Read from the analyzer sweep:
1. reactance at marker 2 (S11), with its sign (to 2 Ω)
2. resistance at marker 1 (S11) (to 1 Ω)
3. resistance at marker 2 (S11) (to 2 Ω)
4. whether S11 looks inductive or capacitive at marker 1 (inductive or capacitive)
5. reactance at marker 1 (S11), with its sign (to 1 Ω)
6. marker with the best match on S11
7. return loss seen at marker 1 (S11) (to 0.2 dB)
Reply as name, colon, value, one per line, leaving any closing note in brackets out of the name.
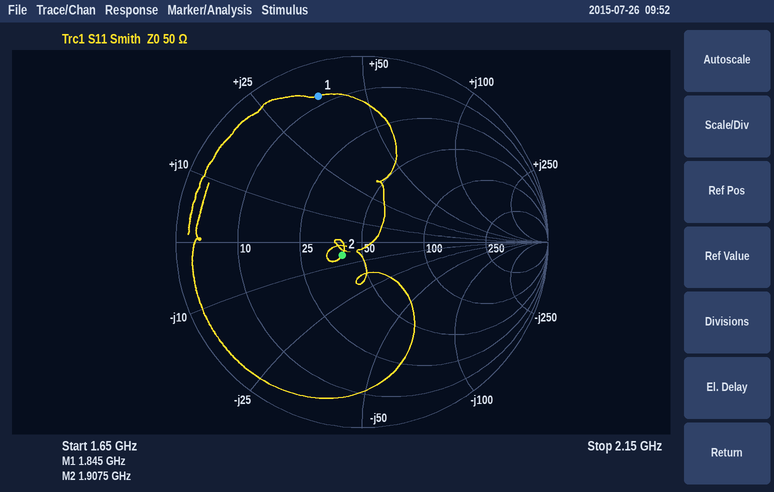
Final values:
reactance at marker 2 (S11), with its sign: -6 Ω
resistance at marker 1 (S11): 8 Ω
resistance at marker 2 (S11): 40 Ω
whether S11 looks inductive or capacitive at marker 1: inductive
reactance at marker 1 (S11), with its sign: +37 Ω
marker with the best match on S11: marker 2
return loss seen at marker 1 (S11): 1.8 dB
